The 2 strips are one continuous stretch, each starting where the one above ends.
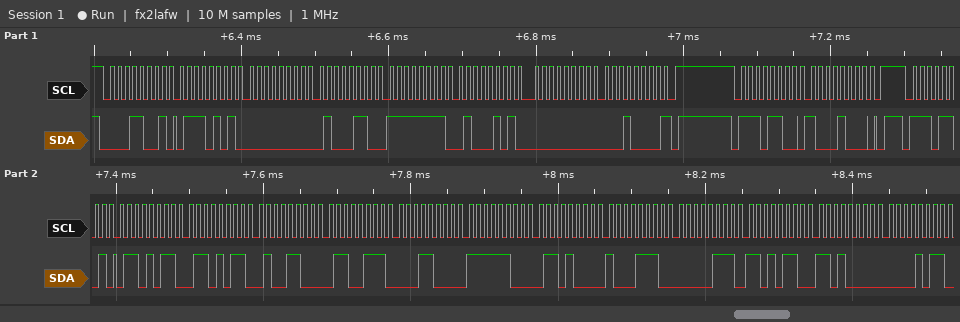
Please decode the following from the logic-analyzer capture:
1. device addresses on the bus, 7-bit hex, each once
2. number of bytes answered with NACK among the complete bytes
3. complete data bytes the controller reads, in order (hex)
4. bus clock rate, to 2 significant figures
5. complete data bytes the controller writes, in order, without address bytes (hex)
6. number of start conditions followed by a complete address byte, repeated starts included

0x0C 0x76
1
75 00 46 FF 45 00 10 6B 6B 4C 67 18 FC 68 8E 07 D6 D0 0B
100 kHz
88
3
